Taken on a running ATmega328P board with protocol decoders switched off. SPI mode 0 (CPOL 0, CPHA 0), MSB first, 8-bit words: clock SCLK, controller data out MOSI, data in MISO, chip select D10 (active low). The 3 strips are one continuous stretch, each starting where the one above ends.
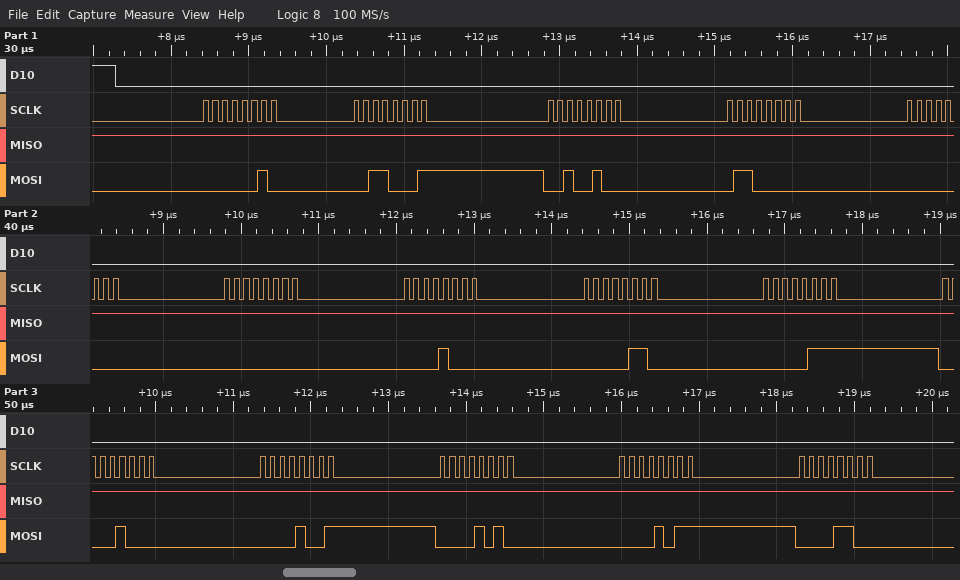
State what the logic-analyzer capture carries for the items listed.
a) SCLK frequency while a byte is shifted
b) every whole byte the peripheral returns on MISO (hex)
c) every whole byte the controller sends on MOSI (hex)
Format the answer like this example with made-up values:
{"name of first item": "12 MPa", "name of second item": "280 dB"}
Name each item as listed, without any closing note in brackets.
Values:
{"SCLK frequency while a byte is shifted": "8 MHz", "every whole byte the peripheral returns on MISO": "FF FF FF FF FF FF FF FF FF FF FF FF FF FF", "every whole byte the controller sends on MOSI": "02 31 24 60 00 00 08 06 07 08 09 0A 0B 0C"}
